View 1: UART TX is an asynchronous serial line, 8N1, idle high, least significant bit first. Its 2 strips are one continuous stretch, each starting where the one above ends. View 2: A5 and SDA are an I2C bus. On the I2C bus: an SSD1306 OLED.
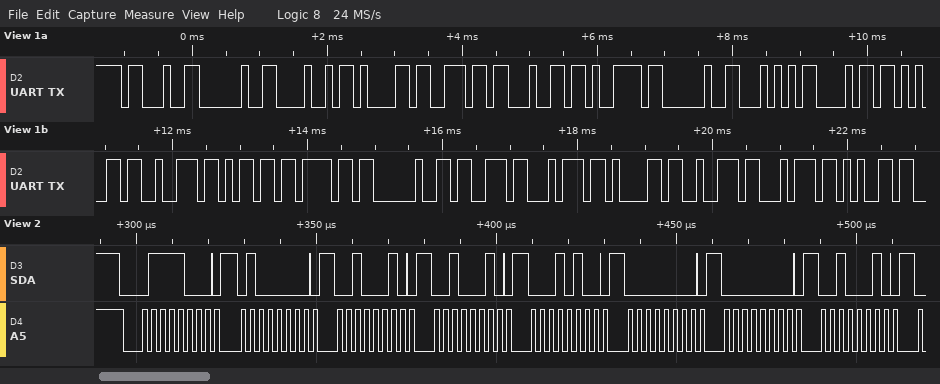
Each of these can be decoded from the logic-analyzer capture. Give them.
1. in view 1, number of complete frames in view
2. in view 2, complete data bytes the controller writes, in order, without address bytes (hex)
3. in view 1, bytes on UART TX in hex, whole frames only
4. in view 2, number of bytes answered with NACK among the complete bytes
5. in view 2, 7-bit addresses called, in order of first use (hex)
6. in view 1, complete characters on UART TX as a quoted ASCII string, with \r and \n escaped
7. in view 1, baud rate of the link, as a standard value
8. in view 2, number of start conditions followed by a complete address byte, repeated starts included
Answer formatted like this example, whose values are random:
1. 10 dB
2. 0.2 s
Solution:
1. 21
2. 40 22 22 14 00 00 22
3. 23 20 48 61 6E 64 79 20 54 68 65 72 6D 6F 20 73 74 61 72 74 65
4. 0
5. 0x3C
6. "# Handy Thermo starte"
7. 9600 baud
8. 1
